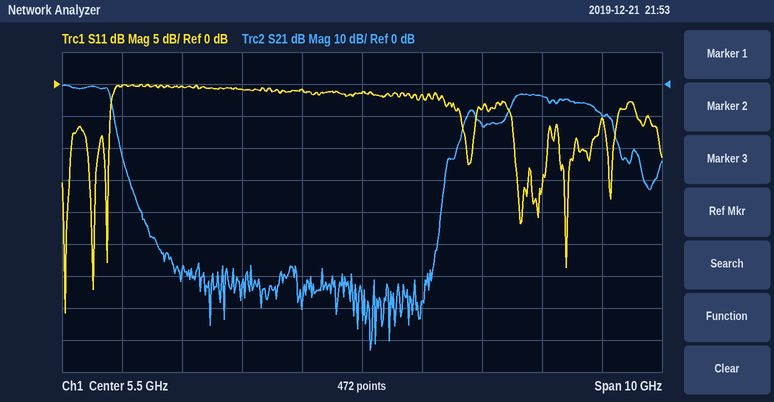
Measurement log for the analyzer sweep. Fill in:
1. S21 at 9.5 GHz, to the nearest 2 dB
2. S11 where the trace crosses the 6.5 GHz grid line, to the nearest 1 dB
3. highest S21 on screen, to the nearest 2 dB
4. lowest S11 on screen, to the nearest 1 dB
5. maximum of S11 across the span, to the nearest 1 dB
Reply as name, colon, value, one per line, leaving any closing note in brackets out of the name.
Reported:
S21 at 9.5 GHz, to the nearest 2 dB: -10 dB
S11 where the trace crosses the 6.5 GHz grid line, to the nearest 1 dB: -2 dB
highest S21 on screen, to the nearest 2 dB: 0 dB
lowest S11 on screen, to the nearest 1 dB: -36 dB
maximum of S11 across the span, to the nearest 1 dB: 0 dB
